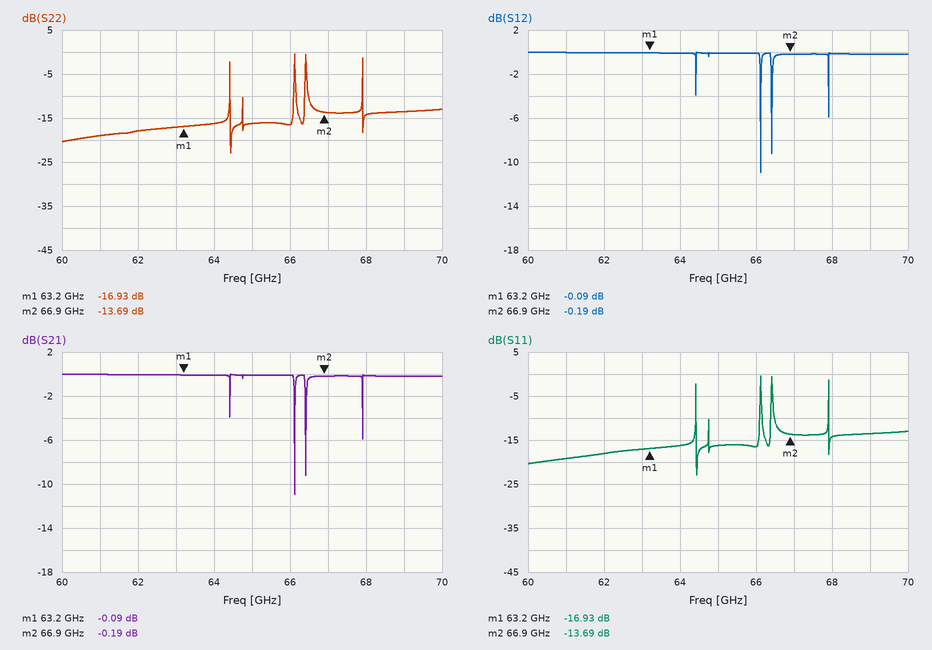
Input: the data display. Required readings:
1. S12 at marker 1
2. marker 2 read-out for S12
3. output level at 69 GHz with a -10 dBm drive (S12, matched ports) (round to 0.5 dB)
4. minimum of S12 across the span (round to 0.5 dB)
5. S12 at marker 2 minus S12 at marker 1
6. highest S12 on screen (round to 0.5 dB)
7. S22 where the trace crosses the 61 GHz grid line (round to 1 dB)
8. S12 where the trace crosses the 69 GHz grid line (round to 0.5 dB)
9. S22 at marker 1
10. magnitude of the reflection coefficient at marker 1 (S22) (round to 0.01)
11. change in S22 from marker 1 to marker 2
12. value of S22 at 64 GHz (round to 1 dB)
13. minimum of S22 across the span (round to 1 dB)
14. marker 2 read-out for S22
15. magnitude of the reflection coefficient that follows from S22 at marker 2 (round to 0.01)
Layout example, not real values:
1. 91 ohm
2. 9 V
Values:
1. -0.09 dB
2. -0.19 dB
3. -10.0 dBm
4. -11.0 dB
5. -0.10 dB
6. 0.0 dB
7. -19 dB
8. 0.0 dB
9. -16.93 dB
10. 0.14
11. 3.24 dB
12. -16 dB
13. -23 dB
14. -13.69 dB
15. 0.21
